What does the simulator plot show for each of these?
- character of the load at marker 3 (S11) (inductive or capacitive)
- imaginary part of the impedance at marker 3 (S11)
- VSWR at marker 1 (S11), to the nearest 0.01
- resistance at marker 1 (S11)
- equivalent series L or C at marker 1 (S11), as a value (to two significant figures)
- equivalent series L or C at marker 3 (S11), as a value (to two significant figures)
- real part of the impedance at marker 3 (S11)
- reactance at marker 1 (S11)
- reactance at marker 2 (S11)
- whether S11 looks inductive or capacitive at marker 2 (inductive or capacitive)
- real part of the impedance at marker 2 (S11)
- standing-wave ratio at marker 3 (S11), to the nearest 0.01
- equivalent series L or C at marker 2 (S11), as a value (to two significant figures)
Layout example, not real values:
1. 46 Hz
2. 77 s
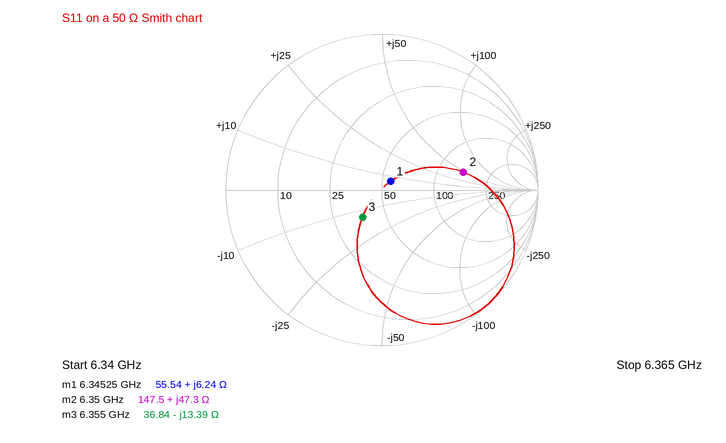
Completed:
1. capacitive
2. -13.39 Ω
3. 1.17
4. 55.54 Ω
5. 160 pH
6. 1.9 pF
7. 36.84 Ω
8. +6.24 Ω
9. +47.3 Ω
10. inductive
11. 147.5 Ω
12. 1.54
13. 1.2 nH
